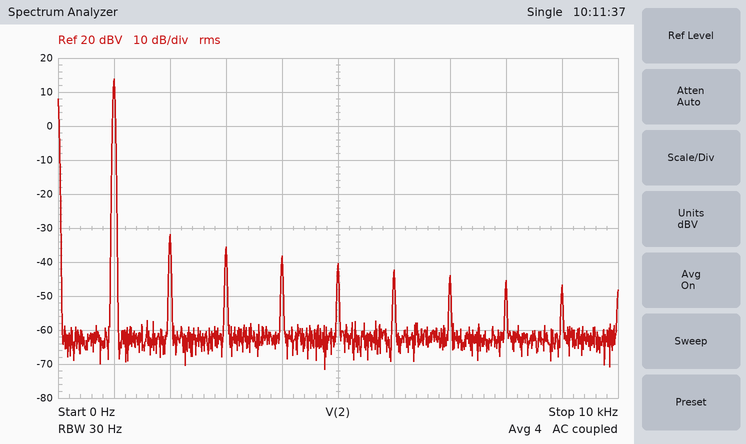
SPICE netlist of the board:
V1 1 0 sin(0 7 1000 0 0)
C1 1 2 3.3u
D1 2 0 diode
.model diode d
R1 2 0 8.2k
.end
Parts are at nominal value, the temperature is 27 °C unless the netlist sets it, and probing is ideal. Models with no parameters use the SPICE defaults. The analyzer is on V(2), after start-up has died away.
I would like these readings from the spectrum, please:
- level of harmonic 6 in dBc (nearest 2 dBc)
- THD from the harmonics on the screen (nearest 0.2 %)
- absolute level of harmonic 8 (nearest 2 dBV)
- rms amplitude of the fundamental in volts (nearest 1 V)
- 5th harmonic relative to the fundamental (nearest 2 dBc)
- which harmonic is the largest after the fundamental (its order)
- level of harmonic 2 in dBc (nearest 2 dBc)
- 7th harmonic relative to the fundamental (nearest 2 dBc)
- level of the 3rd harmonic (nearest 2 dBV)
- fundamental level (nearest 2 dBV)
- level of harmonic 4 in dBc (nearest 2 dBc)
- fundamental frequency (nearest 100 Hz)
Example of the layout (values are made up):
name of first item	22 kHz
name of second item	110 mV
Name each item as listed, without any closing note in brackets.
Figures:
level of harmonic 6 in dBc	-56 dBc
THD from the harmonics on the screen	0.8 %
absolute level of harmonic 8	-46 dBV
rms amplitude of the fundamental in volts	5 V
5th harmonic relative to the fundamental	-54 dBc
which harmonic is the largest after the fundamental	2
level of harmonic 2 in dBc	-46 dBc
7th harmonic relative to the fundamental	-58 dBc
level of the 3rd harmonic	-36 dBV
fundamental level	14 dBV
level of harmonic 4 in dBc	-52 dBc
fundamental frequency	1.0 kHz
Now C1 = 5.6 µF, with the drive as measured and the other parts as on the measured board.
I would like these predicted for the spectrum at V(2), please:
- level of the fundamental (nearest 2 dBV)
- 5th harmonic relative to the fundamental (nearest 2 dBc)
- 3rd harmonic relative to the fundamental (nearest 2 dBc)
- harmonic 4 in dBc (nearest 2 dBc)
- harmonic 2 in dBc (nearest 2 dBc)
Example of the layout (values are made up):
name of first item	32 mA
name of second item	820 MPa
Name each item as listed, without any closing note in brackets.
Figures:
level of the fundamental	14 dBV
5th harmonic relative to the fundamental	-58 dBc
3rd harmonic relative to the fundamental	-54 dBc
harmonic 4 in dBc	-56 dBc
harmonic 2 in dBc	-50 dBc
